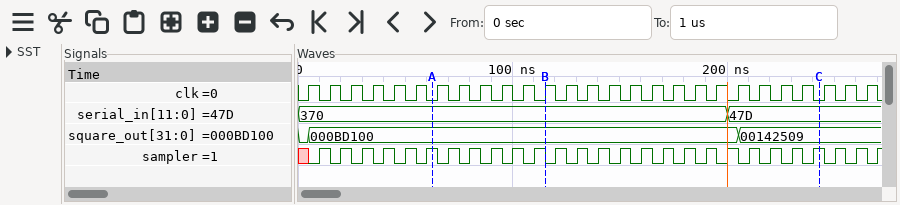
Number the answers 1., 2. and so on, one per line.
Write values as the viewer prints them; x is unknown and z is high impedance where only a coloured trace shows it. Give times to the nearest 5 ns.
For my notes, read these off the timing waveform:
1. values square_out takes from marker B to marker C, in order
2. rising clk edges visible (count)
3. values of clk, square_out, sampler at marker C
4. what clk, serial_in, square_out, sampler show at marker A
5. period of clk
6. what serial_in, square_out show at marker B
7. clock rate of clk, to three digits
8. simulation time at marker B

1. 000BD100, 00142509
2. 27
3. clk=0, square_out=00142509, sampler=1
4. clk=0, serial_in=370, square_out=000BD100, sampler=1
5. 10 ns
6. serial_in=370, square_out=000BD100
7. 100 MHz
8. 115 ns
